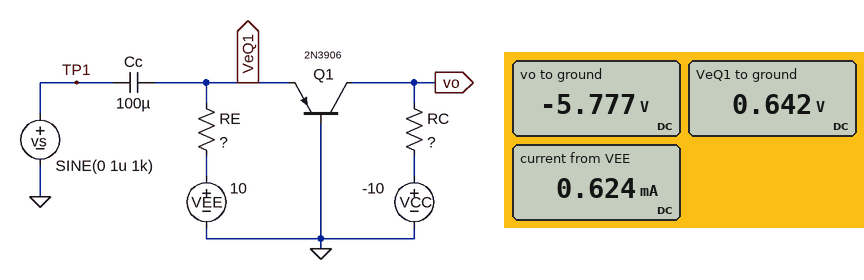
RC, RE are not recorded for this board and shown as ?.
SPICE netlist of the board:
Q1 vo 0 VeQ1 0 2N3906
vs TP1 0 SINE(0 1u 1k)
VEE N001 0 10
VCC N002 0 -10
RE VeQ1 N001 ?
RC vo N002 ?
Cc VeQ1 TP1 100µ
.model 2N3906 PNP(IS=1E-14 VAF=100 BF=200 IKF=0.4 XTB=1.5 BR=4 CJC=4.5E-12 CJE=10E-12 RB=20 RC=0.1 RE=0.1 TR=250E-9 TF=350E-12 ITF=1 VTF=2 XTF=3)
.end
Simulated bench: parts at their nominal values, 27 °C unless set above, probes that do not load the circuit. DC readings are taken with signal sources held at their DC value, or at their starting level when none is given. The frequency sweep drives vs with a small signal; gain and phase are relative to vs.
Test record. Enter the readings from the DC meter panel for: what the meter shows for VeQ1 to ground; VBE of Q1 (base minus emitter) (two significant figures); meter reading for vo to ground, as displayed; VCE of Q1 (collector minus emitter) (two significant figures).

0.642 V
-640 mV
-5.777 V
-6.4 V
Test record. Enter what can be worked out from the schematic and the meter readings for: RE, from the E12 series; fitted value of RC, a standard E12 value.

15 kΩ
6.8 kΩ
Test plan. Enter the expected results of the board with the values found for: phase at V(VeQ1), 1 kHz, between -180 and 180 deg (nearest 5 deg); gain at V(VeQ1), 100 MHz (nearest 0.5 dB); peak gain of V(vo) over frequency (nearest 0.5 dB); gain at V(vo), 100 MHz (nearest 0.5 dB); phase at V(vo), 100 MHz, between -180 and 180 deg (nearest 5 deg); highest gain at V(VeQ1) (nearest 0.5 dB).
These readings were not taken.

0 deg
0 dB
44.0 dB
21.0 dB
-95 deg
0 dB
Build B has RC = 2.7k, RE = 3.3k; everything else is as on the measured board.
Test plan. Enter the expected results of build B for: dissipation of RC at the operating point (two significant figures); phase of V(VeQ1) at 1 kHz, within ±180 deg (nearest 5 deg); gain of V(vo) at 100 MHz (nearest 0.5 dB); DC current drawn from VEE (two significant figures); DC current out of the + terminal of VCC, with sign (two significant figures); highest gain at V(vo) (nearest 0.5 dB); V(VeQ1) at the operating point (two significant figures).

21 mW
10 deg
25.0 dB
2.8 mA
-2.8 mA
48.5 dB
680 mV
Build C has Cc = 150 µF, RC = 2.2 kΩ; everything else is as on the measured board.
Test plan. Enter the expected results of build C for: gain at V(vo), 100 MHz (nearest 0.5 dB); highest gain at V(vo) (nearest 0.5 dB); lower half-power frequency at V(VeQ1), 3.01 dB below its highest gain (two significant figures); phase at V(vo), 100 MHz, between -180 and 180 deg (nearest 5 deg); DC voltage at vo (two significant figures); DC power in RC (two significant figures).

21.5 dB
34.5 dB
25 Hz
-85 deg
-8.6 V
850 µW
